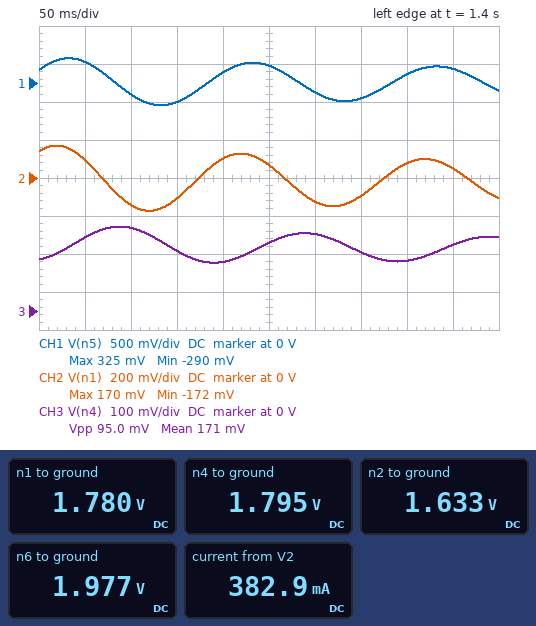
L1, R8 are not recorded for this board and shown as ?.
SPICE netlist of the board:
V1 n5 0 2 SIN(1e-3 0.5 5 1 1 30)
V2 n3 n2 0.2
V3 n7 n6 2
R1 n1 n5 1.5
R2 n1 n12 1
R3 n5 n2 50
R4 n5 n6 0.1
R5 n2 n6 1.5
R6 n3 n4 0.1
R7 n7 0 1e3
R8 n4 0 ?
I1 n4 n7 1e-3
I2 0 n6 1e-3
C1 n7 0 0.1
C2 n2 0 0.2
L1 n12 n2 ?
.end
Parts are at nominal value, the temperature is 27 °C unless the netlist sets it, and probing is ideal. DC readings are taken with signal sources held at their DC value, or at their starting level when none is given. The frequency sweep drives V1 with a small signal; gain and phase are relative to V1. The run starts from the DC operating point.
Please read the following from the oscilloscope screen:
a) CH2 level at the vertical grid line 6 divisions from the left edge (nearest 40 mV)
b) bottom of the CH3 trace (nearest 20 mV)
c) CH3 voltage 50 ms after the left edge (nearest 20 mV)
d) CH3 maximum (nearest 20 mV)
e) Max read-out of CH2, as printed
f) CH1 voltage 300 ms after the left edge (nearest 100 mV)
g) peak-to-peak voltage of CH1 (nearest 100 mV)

-120 mV
120 mV
200 mV
220 mV
170 mV
-100 mV
600 mV
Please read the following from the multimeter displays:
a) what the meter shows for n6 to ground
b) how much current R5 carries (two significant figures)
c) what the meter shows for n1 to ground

1.977 V
230 mA
1.780 V
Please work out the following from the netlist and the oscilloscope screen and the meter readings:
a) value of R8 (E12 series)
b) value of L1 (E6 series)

4.7 Ω
47 mH
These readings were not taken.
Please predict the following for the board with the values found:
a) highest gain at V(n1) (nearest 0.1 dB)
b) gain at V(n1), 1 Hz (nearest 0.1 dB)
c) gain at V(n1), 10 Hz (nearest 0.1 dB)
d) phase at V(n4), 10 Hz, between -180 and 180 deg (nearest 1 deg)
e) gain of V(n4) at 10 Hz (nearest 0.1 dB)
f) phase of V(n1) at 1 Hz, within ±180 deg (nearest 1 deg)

0 dB
-3.7 dB
-2.1 dB
-121 deg
-24.0 dB
-20 deg
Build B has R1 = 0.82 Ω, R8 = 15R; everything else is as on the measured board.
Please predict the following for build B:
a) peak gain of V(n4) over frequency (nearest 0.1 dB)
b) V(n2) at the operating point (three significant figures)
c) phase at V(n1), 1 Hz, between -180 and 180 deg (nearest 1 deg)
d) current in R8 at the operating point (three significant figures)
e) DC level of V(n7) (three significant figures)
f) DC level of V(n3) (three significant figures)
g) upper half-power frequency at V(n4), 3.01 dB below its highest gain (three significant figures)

-0.5 dB
1.88 V
-15 deg
138 mA
3.99 V
2.08 V
1.07 Hz
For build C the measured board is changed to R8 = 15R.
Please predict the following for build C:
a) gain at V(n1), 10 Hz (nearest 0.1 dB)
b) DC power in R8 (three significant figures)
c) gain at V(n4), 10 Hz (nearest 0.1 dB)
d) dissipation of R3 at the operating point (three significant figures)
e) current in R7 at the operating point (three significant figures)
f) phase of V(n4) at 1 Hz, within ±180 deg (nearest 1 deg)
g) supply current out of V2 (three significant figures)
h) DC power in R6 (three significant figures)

-2.1 dB
281 mW
-23.8 dB
349 µW
3.99 mA
-52 deg
138 mA
1.90 mW
